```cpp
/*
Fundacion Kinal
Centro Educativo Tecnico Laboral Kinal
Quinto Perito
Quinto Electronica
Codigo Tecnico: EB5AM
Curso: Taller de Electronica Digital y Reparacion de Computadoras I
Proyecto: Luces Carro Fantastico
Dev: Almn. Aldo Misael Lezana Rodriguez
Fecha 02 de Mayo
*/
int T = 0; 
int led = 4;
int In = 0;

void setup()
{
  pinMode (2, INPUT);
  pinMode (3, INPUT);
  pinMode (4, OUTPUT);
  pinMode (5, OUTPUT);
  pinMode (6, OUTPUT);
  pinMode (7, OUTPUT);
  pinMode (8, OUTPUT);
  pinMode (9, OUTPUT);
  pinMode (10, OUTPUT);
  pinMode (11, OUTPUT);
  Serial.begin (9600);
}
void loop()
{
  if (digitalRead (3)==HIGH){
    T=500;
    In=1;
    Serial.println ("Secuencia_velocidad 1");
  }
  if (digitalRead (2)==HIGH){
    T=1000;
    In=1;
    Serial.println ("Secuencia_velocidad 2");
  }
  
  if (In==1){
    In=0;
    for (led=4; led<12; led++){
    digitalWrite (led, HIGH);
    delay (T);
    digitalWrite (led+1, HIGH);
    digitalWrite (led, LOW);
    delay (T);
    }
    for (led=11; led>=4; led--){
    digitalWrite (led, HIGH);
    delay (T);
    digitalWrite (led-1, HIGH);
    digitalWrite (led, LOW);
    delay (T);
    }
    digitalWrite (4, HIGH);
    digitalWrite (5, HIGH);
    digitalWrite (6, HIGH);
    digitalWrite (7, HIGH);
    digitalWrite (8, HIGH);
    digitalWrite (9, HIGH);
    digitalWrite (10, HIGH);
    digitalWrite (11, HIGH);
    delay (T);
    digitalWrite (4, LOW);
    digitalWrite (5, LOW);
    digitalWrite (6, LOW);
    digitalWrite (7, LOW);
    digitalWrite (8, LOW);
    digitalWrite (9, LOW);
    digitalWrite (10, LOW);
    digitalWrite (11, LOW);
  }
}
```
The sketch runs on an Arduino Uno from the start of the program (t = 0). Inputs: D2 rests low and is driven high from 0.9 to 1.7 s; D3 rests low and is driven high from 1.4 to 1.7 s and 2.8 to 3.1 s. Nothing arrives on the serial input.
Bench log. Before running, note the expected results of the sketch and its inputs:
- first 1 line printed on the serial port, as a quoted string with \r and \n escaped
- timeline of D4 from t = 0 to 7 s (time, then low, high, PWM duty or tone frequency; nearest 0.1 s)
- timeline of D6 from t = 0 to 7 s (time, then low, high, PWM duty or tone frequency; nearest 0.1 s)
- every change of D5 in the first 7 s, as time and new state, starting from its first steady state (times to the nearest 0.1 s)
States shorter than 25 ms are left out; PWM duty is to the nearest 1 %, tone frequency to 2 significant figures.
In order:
"Secuencia_velocidad 2\r\n"
0 s low; 0.9 s high; 1.9 s low
0 s low; 3.9 s high; 5.9 s low
0 s low; 1.9 s high; 3.9 s low
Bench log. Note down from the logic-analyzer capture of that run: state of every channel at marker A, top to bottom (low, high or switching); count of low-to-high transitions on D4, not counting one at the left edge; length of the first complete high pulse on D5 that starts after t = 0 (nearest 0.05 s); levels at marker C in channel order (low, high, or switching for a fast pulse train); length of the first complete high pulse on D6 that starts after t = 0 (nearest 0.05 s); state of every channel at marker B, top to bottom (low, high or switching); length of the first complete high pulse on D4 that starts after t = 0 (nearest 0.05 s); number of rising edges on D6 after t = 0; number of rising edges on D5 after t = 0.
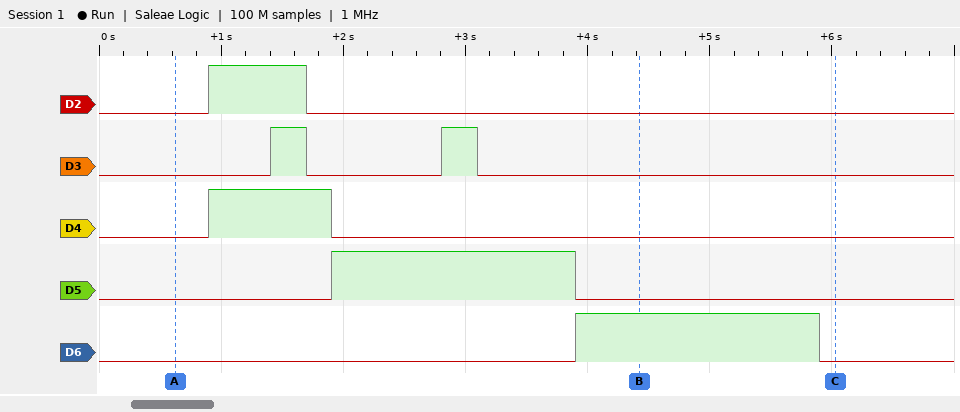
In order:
D2 low, D3 low, D4 low, D5 low, D6 low
1
2.00 s
D2 low, D3 low, D4 low, D5 low, D6 low
2.00 s
D2 low, D3 low, D4 low, D5 low, D6 high
1.00 s
1
1
